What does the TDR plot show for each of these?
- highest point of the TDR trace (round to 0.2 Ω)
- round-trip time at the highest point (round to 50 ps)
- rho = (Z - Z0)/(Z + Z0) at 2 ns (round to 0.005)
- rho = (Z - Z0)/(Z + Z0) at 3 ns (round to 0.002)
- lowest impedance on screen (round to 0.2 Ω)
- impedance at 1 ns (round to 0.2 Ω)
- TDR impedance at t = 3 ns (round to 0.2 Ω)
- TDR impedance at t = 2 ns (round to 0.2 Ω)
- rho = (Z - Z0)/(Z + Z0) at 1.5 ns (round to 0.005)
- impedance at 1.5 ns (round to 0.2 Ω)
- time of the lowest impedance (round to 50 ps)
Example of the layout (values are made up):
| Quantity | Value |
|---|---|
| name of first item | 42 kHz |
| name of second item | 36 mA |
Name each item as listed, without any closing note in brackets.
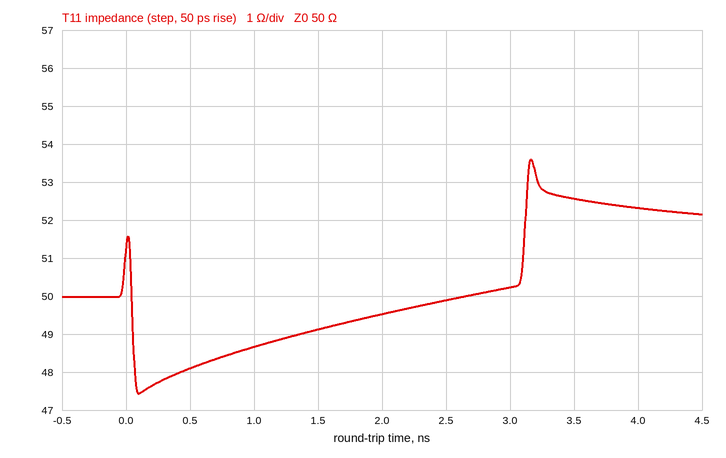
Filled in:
| Quantity | Value |
|---|---|
| highest point of the TDR trace | 53.6 Ω |
| round-trip time at the highest point | 3.15 ns |
| rho = (Z - Z0)/(Z + Z0) at 2 ns | -0.005 |
| rho = (Z - Z0)/(Z + Z0) at 3 ns | +0.002 |
| lowest impedance on screen | 47.4 Ω |
| impedance at 1 ns | 48.6 Ω |
| TDR impedance at t = 3 ns | 50.2 Ω |
| TDR impedance at t = 2 ns | 49.6 Ω |
| rho = (Z - Z0)/(Z + Z0) at 1.5 ns | -0.010 |
| impedance at 1.5 ns | 49.2 Ω |
| time of the lowest impedance | 100 ps |
